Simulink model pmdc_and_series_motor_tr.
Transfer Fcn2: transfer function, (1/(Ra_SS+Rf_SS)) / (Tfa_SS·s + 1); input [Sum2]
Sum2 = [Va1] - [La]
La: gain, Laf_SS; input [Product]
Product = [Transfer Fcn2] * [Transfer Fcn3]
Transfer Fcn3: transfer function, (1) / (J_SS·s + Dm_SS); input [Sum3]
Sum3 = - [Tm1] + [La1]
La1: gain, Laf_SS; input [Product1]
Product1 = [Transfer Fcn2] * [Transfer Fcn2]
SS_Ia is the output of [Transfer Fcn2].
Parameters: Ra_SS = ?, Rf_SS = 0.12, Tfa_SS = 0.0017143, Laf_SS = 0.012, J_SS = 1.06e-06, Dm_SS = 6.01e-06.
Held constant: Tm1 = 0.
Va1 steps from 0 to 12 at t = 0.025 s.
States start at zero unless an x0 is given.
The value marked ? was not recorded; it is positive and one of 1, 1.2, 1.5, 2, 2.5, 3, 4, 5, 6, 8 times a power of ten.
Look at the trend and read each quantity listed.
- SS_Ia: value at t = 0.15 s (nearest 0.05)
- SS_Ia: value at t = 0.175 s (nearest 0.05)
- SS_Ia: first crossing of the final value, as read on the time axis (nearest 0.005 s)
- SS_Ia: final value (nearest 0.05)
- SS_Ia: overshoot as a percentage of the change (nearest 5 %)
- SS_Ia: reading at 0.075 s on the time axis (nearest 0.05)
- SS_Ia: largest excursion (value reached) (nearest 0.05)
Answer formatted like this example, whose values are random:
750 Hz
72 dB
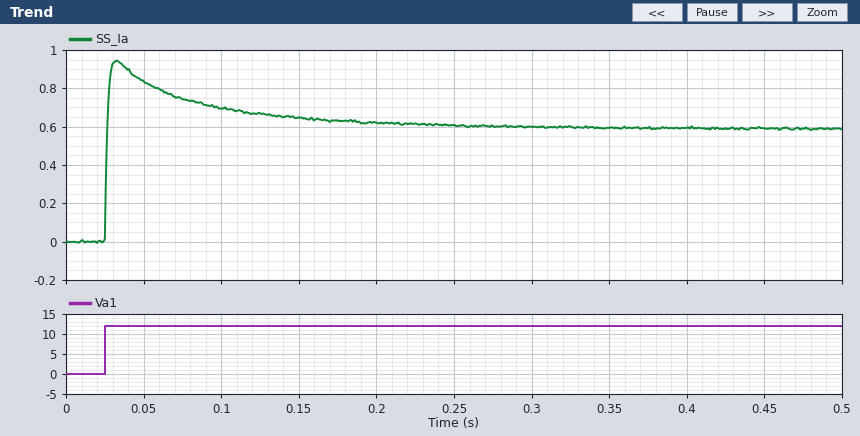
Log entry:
0.65
0.65
0.025 s
0.60
60 %
0.75
0.95
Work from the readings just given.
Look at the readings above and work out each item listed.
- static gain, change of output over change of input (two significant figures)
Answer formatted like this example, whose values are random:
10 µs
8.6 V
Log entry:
0.050
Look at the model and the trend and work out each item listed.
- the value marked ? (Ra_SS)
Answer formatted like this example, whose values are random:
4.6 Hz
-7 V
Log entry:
12
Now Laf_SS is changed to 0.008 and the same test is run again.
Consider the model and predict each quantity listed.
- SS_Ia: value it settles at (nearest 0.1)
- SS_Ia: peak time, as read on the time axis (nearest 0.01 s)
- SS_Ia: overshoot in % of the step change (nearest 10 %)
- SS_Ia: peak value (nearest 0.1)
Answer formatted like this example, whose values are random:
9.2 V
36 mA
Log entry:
0.7
0.03 s
40 %
1.0
